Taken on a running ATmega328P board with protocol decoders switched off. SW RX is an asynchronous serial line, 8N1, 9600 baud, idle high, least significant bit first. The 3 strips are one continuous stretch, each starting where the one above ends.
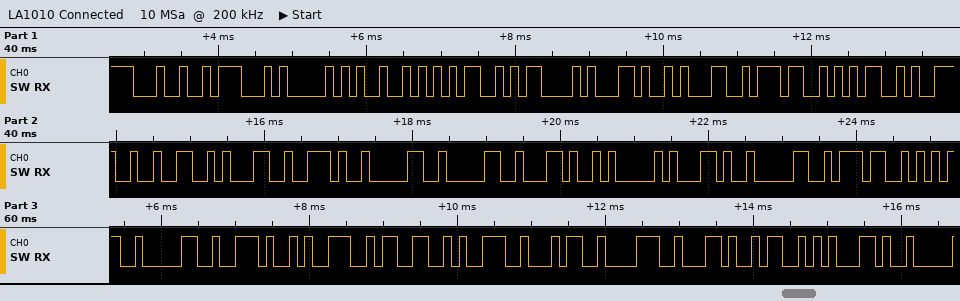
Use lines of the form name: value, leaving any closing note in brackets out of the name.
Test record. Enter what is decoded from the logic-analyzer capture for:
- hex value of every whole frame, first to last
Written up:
hex value of every whole frame, first to last: 24 47 50 52 4D 43 2C 31 37 35 39 32 31 2E 30 30 2C 41 2C 30 37 35 30 2E 39 33 39 34 38 2C 53 2C
